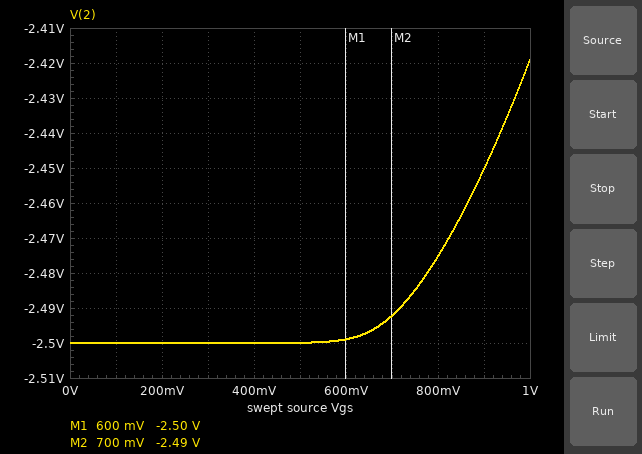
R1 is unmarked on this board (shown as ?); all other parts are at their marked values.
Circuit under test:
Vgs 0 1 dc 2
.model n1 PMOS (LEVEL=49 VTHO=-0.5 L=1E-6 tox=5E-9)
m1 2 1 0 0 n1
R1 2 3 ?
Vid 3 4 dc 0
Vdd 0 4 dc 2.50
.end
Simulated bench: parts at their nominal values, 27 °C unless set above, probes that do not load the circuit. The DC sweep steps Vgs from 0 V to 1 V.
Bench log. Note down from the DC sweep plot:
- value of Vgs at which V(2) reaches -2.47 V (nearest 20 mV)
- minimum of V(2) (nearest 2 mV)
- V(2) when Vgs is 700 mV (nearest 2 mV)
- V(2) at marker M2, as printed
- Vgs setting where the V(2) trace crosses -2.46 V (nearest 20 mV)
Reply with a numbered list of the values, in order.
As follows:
1. 820 mV
2. -2.500 V
3. -2.492 V
4. -2.49 V
5. 860 mV
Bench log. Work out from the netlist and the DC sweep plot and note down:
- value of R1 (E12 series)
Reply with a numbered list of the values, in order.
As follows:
1. 2.2 kΩ
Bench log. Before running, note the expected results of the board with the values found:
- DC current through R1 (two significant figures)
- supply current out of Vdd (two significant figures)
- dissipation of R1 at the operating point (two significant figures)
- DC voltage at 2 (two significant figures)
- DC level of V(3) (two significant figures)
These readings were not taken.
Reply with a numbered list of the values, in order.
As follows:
1. 280 µA
2. 280 µA
3. 180 µW
4. -1.9 V
5. -2.5 V
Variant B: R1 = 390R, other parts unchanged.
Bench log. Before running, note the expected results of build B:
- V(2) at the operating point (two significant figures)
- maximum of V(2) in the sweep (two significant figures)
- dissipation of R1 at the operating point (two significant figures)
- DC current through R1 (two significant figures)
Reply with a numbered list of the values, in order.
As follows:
1. -2.4 V
2. -2.5 V
3. 32 µW
4. 290 µA
